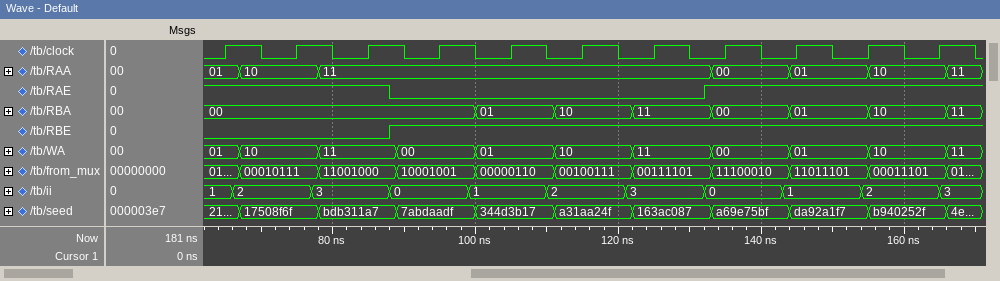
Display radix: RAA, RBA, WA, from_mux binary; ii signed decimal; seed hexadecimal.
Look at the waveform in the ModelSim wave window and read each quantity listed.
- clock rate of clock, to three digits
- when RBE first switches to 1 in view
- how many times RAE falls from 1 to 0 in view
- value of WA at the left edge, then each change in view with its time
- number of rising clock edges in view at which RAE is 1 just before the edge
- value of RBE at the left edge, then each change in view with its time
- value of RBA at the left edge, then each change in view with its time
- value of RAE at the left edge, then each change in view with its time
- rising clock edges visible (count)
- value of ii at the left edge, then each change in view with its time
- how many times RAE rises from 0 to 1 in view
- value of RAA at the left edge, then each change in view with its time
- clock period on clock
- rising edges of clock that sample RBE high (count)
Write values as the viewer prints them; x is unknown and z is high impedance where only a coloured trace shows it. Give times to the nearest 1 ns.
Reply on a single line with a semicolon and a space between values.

100 MHz; 88 ns; 1; 01, 10 at 67 ns, 11 at 78 ns, 00 at 89 ns, 01 at 100 ns, 10 at 111 ns, 11 at 122 ns, 00 at 133 ns, 01 at 144 ns, 10 at 155 ns, 11 at 166 ns; 7; 0, 1 at 88 ns; 00, 01 at 100 ns, 10 at 111 ns, 11 at 122 ns, 00 at 133 ns, 01 at 144 ns, 10 at 155 ns, 11 at 166 ns; 1, 0 at 88 ns, 1 at 132 ns; 11; 1, 2 at 66 ns, 3 at 77 ns, 0 at 88 ns, 1 at 99 ns, 2 at 110 ns, 3 at 121 ns, 0 at 132 ns, 1 at 143 ns, 2 at 154 ns, 3 at 165 ns; 1; 01, 10 at 67 ns, 11 at 78 ns, 00 at 133 ns, 01 at 144 ns, 10 at 155 ns, 11 at 166 ns; 10 ns; 8
